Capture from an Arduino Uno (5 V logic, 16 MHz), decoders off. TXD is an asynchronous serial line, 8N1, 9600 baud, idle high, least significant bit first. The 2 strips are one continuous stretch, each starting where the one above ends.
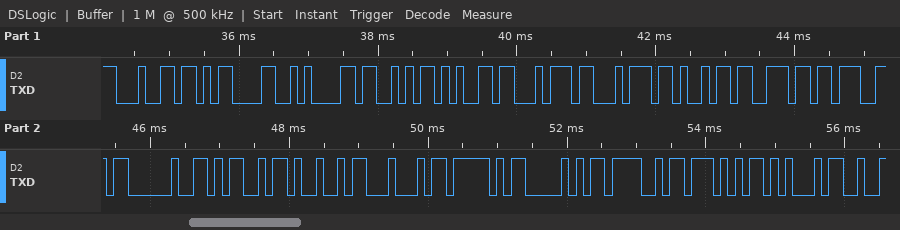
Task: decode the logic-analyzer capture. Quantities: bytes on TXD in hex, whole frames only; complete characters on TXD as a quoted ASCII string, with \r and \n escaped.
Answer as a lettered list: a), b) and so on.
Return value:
a) 64 0D 0A 53 65 74 74 69 6E 67 20 4D 49 44 5F 50 4F 57 45
b) "d\r\nSetting MID_POWE"
